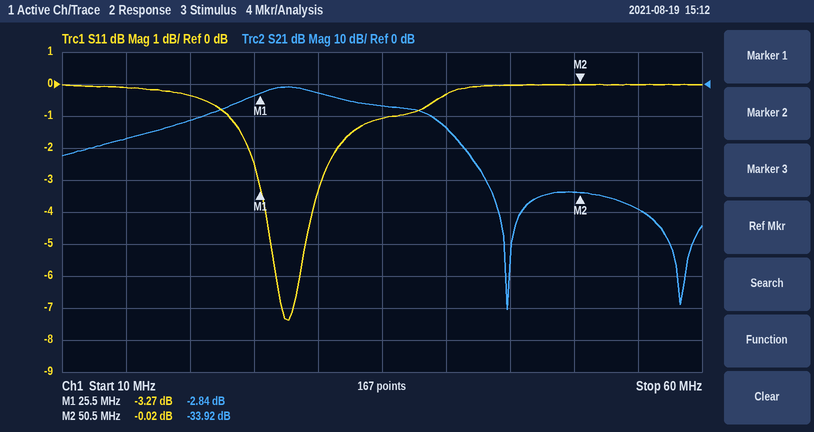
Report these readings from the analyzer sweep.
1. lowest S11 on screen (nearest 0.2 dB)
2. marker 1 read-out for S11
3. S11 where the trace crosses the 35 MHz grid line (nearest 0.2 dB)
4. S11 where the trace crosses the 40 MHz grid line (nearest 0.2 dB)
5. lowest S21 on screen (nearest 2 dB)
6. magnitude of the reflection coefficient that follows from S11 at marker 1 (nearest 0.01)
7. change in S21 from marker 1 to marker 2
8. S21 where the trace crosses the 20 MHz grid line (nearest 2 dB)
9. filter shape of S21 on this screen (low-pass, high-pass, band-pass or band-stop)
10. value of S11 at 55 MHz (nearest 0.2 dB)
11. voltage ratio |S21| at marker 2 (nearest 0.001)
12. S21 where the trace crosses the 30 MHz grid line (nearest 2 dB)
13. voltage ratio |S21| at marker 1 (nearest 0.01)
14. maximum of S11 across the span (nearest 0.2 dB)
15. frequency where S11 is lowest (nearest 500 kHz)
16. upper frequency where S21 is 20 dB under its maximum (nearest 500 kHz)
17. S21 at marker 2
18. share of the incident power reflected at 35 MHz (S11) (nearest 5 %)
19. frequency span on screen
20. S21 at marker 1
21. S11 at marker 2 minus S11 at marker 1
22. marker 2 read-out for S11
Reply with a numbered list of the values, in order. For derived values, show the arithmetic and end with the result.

1. -7.4 dB
2. -3.27 dB
3. -1.0 dB
4. -0.4 dB
5. -70 dB
6. 10^(-3.27/20) ≈ 0.69
7. -33.92 − (-2.84) = -31.08 dB
8. -12 dB
9. band-pass
10. 0.0 dB
11. 10^(-33.92/20) ≈ 0.020
12. -2 dB
13. 10^(-2.84/20) ≈ 0.72
14. 0.0 dB
15. 27.5 MHz
16. 41.5 MHz
17. -33.92 dB
18. 10^(-1/10) ≈ 79.4 %, so 80 % to the nearest 5 %
19. 50 MHz
20. -2.84 dB
21. -0.02 − (-3.27) = 3.25 dB
22. -0.02 dB
